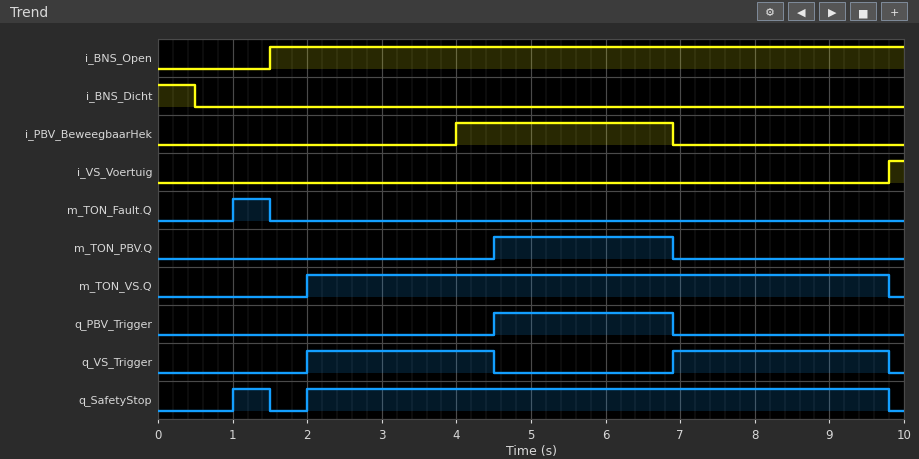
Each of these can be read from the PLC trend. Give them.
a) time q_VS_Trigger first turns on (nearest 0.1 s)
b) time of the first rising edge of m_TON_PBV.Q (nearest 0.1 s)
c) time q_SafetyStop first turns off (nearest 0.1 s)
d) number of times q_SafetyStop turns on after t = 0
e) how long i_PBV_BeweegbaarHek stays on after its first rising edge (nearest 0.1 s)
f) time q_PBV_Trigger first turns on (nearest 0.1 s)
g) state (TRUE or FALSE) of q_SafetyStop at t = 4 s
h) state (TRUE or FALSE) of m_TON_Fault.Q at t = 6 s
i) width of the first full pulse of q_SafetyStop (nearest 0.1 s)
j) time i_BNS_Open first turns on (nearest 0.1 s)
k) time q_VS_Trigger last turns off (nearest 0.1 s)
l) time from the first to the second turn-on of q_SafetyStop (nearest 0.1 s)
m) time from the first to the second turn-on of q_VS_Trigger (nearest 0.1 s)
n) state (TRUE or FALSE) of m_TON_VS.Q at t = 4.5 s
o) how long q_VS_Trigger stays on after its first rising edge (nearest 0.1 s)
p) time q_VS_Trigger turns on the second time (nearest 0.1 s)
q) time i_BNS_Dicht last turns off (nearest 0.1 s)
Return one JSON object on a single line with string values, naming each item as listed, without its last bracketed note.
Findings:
{"time q_VS_Trigger first turns on": "2.0 s", "time of the first rising edge of m_TON_PBV.Q": "4.5 s", "time q_SafetyStop first turns off": "1.5 s", "number of times q_SafetyStop turns on after t = 0": "2", "how long i_PBV_BeweegbaarHek stays on after its first rising edge": "2.9 s", "time q_PBV_Trigger first turns on": "4.5 s", "state (TRUE or FALSE) of q_SafetyStop at t = 4 s": "TRUE", "state (TRUE or FALSE) of m_TON_Fault.Q at t = 6 s": "FALSE", "width of the first full pulse of q_SafetyStop": "0.5 s", "time i_BNS_Open first turns on": "1.5 s", "time q_VS_Trigger last turns off": "9.8 s", "time from the first to the second turn-on of q_SafetyStop": "1.0 s", "time from the first to the second turn-on of q_VS_Trigger": "4.9 s", "state (TRUE or FALSE) of m_TON_VS.Q at t = 4.5 s": "TRUE", "how long q_VS_Trigger stays on after its first rising edge": "2.5 s", "time q_VS_Trigger turns on the second time": "6.9 s", "time i_BNS_Dicht last turns off": "0.5 s"}
